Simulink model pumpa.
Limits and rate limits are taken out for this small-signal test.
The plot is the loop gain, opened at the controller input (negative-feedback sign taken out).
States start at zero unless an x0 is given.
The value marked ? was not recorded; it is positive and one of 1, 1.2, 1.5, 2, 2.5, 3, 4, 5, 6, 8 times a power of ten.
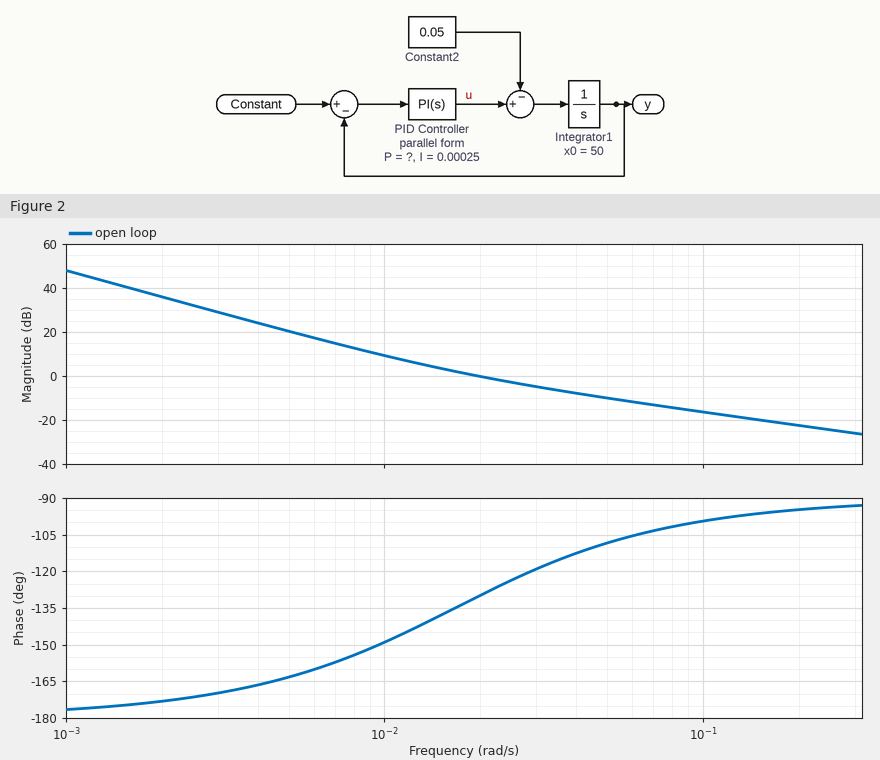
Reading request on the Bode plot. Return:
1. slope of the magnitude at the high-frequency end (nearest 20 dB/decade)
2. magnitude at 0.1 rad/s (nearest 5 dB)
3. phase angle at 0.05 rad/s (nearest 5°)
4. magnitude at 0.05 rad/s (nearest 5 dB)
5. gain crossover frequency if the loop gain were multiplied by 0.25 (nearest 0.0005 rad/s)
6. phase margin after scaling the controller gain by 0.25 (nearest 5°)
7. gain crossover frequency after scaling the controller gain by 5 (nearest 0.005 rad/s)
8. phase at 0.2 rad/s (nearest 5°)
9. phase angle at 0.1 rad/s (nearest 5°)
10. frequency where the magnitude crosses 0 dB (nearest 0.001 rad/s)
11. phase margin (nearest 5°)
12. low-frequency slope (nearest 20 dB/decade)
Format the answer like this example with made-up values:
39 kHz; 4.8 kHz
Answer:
-20 dB/decade; -15 dB; -110°; -10 dB; 0.0085 rad/s; 25°; 0.075 rad/s; -95°; -100°; 0.020 rad/s; 50°; -40 dB/decade
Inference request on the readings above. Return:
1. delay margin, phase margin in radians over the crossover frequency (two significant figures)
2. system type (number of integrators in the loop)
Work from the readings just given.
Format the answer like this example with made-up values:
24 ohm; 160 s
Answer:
44 s; 2
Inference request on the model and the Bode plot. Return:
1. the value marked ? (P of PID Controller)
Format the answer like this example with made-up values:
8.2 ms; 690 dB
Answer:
0.015
